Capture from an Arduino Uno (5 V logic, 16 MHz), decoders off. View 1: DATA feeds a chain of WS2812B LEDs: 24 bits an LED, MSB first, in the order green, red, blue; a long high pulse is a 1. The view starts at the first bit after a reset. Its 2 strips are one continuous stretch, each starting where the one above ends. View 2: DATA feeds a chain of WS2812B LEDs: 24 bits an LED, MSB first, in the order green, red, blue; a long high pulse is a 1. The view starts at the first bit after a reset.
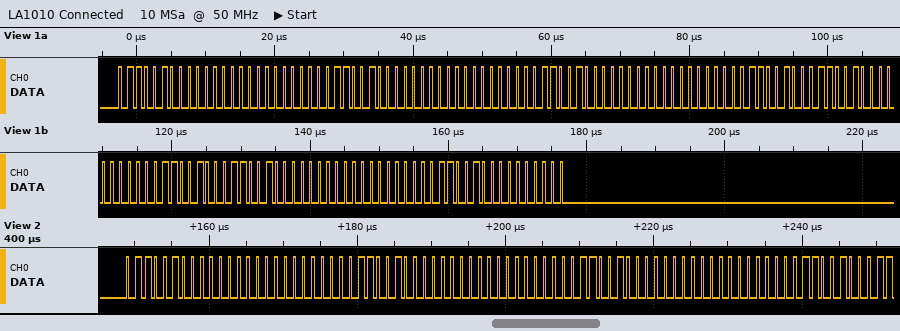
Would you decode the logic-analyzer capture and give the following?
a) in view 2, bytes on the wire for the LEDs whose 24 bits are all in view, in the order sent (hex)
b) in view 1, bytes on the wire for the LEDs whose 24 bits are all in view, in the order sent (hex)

64 00 00 64 00 00 64 00 00
64 00 00 64 00 00 64 00 00 64 64 00 64 64 00 00 64 00
